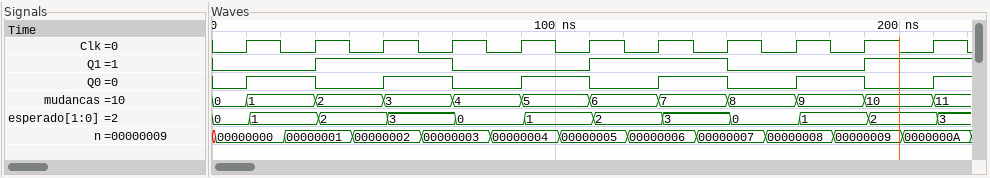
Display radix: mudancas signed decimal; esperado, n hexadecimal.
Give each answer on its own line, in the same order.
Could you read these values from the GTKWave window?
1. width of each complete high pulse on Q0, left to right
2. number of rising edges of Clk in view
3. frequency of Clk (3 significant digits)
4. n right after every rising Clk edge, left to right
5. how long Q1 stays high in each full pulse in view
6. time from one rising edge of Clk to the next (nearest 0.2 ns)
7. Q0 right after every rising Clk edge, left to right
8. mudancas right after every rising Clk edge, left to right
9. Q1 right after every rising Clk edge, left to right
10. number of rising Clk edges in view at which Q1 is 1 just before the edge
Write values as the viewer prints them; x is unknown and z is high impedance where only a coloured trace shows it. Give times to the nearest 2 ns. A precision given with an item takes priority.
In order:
20 ns, 20 ns, 20 ns, 20 ns, 20 ns
11
50.0 MHz
00000000, 00000001, 00000002, 00000003, 00000004, 00000005, 00000006, 00000007, 00000008, 00000009, 0000000A
40 ns, 40 ns
20 ns
1 0 1 0 1 0 1 0 1 0 1
1, 2, 3, 4, 5, 6, 7, 8, 9, 10, 11
0 1 1 0 0 1 1 0 0 1 1
5
